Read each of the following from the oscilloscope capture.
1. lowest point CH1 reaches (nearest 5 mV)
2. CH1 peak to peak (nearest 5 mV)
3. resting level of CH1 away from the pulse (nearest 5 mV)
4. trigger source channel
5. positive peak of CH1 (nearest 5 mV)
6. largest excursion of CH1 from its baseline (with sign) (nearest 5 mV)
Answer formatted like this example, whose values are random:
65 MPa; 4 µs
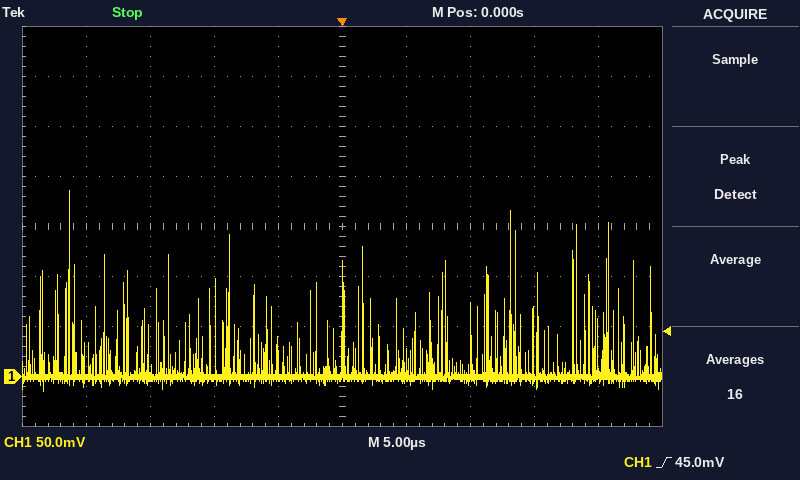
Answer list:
-15 mV; 200 mV; 0 mV; CH1; 185 mV; +185 mV
